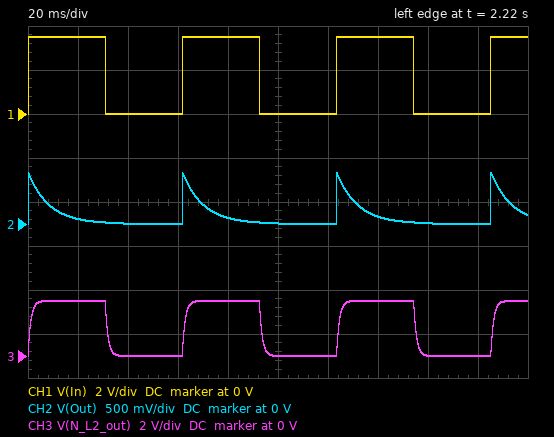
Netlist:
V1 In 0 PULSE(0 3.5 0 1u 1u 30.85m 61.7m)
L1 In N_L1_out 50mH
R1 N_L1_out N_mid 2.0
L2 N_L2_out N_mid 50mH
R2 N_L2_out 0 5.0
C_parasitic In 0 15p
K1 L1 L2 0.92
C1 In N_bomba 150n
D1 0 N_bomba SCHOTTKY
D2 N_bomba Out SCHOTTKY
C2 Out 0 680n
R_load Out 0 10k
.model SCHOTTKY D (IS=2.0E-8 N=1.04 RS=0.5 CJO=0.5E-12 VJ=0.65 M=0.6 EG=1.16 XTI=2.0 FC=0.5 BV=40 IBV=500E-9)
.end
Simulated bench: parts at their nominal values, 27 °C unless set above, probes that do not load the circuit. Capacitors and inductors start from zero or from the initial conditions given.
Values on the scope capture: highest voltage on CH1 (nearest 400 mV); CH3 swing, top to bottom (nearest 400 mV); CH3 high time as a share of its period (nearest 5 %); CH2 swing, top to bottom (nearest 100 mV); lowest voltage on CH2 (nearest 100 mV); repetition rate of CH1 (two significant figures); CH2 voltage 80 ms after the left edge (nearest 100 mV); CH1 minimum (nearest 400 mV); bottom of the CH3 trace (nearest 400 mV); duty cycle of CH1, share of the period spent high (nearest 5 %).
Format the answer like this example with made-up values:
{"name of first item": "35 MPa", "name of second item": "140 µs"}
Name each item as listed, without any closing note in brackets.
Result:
{"highest voltage on CH1": "3.6 V", "CH3 swing, top to bottom": "2.4 V", "CH3 high time as a share of its period": "50 %", "CH2 swing, top to bottom": "600 mV", "lowest voltage on CH2": "0 V", "repetition rate of CH1": "16 Hz", "CH2 voltage 80 ms after the left edge": "100 mV", "CH1 minimum": "0 V", "bottom of the CH3 trace": "0 V", "duty cycle of CH1, share of the period spent high": "50 %"}
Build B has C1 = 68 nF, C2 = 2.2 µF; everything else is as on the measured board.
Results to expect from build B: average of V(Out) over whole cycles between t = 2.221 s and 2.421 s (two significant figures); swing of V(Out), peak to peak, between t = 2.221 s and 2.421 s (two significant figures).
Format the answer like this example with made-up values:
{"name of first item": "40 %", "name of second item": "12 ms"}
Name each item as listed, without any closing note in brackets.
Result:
{"average of V(Out) over whole cycles between t = 2.221 s and 2.421 s": "37 mV", "swing of V(Out), peak to peak, between t = 2.221 s and 2.421 s": "98 mV"}
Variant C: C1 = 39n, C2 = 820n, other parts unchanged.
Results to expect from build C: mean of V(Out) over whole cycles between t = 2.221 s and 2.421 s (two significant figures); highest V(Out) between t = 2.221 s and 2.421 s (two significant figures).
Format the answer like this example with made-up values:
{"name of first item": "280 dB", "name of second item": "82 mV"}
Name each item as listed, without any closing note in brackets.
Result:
{"mean of V(Out) over whole cycles between t = 2.221 s and 2.421 s": "22 mV", "highest V(Out) between t = 2.221 s and 2.421 s": "150 mV"}
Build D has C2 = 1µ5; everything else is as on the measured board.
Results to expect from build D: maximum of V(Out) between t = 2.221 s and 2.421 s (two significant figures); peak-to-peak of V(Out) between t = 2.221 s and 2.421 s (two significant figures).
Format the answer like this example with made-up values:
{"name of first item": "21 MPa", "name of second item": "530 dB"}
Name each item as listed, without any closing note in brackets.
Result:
{"maximum of V(Out) between t = 2.221 s and 2.421 s": "300 mV", "peak-to-peak of V(Out) between t = 2.221 s and 2.421 s": "290 mV"}
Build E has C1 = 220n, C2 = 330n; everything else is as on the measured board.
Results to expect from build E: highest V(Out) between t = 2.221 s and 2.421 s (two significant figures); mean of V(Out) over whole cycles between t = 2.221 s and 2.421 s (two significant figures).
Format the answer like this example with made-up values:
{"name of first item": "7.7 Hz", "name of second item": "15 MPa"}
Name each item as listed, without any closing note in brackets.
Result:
{"highest V(Out) between t = 2.221 s and 2.421 s": "1.3 V", "mean of V(Out) over whole cycles between t = 2.221 s and 2.421 s": "120 mV"}
